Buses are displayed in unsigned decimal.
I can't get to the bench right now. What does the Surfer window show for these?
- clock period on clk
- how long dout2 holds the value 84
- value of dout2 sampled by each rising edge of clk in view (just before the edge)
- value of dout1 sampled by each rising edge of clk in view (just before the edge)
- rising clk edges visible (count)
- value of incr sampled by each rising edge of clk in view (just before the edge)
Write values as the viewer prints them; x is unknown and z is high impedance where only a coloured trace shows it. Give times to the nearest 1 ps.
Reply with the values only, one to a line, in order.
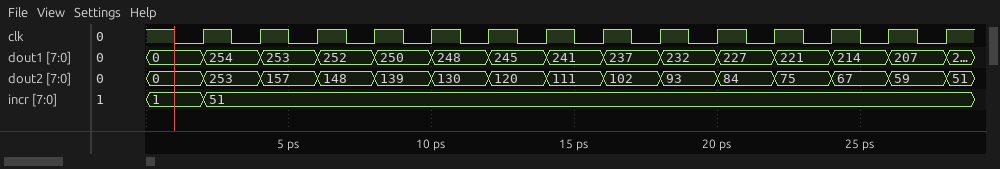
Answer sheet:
2 ps
2 ps
0, 253, 157, 148, 139, 130, 120, 111, 102, 93, 84, 75, 67, 59
0, 254, 253, 252, 250, 248, 245, 241, 237, 232, 227, 221, 214, 207
14
1, 51, 51, 51, 51, 51, 51, 51, 51, 51, 51, 51, 51, 51
